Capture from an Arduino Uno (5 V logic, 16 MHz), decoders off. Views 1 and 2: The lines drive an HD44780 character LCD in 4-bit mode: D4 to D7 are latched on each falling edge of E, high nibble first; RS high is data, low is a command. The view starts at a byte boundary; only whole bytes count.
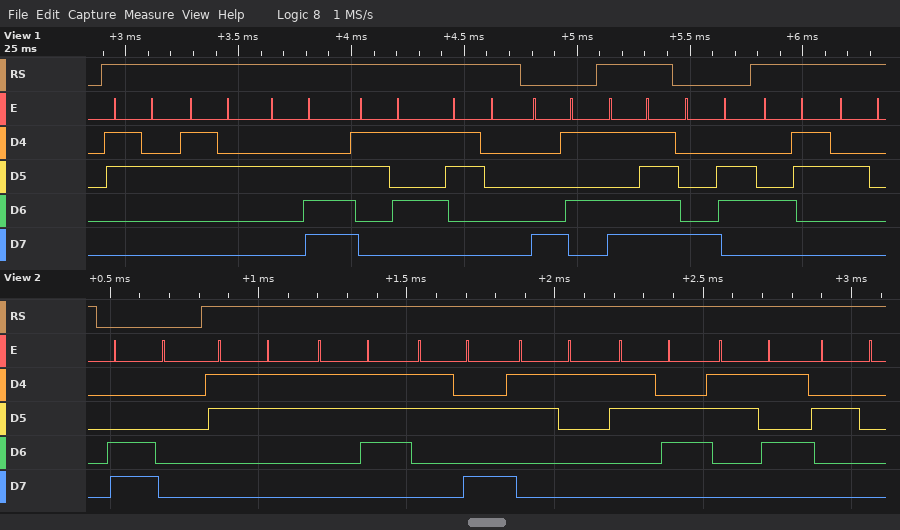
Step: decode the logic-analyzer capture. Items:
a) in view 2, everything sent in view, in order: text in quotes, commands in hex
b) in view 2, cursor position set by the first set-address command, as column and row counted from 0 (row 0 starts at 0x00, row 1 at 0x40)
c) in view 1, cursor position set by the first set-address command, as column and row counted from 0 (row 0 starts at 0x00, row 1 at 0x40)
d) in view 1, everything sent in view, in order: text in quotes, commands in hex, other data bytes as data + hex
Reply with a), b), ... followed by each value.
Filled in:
a) 0xC0 "37:165 "
b) column 0, row 1
c) column 5, row 0
d) "22.50" 0x85 data DF 0x86 "C "
